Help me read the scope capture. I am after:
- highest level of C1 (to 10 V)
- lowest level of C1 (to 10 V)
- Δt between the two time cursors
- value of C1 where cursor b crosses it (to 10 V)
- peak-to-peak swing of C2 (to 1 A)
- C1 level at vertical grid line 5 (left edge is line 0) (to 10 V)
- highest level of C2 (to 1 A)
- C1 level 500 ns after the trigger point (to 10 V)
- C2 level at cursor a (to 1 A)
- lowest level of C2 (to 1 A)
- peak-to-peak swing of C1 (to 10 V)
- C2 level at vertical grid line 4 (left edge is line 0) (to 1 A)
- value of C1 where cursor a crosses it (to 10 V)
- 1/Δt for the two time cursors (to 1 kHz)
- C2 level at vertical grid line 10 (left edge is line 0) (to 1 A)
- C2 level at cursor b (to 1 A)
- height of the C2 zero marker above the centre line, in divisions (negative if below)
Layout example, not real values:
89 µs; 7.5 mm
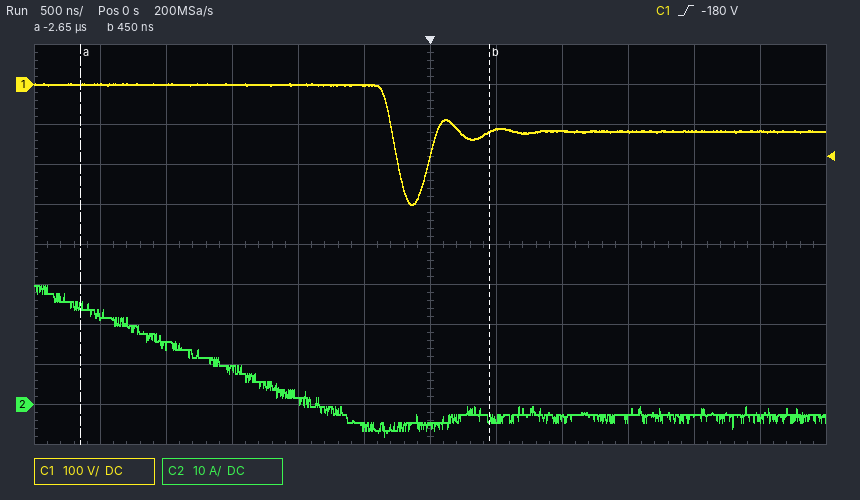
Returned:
0 V; -300 V; 3.10 µs; -120 V; 38 A; 0 V; 30 A; -110 V; 25 A; -8 A; 300 V; 1 A; 0 V; 323 kHz; -3 A; -3 A; -4.0 div
